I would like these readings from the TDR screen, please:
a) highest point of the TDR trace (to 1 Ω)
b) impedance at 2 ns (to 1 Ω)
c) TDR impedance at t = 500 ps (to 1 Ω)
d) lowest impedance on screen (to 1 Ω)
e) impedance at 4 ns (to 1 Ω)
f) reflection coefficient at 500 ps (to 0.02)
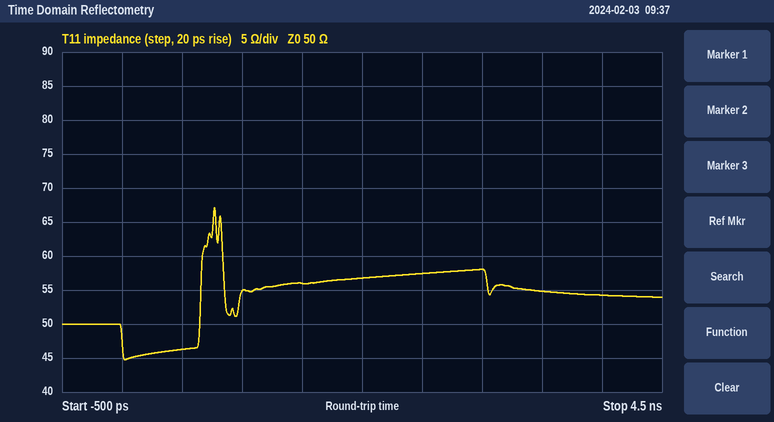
67 Ω
57 Ω
46 Ω
45 Ω
54 Ω
-0.04
